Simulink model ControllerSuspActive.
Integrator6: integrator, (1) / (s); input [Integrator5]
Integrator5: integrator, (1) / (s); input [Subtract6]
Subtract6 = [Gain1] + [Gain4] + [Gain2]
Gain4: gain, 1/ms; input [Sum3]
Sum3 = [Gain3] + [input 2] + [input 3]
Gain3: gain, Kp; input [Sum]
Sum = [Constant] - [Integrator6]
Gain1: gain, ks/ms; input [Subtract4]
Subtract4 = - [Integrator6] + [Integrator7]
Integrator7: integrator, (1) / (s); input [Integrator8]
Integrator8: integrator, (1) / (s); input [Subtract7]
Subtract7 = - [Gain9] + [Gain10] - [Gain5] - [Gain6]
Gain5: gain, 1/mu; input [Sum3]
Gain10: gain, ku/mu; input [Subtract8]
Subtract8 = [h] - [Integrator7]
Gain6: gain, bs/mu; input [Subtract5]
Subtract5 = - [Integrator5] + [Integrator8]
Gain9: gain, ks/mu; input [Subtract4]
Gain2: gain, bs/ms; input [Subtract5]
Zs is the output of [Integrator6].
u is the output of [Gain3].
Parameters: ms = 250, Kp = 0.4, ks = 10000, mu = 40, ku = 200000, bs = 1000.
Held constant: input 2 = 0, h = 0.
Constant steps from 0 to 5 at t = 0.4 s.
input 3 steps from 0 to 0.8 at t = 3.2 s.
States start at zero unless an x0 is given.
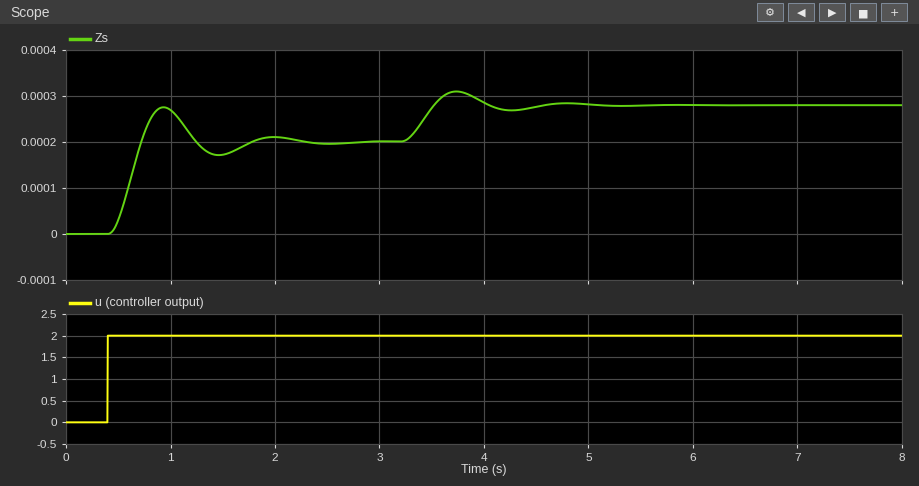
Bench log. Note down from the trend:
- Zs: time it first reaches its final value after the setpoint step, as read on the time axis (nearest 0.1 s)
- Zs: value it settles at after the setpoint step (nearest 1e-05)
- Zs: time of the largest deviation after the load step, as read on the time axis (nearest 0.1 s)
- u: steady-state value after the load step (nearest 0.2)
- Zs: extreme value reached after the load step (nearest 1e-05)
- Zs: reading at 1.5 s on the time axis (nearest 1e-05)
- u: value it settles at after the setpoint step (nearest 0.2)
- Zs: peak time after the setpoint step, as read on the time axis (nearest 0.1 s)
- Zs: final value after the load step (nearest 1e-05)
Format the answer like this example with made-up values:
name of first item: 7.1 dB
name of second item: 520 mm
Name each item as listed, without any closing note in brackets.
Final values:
Zs: time it first reaches its final value after the setpoint step, as read on the time axis: 0.7 s
Zs: value it settles at after the setpoint step: 0.00020
Zs: time of the largest deviation after the load step, as read on the time axis: 3.7 s
u: steady-state value after the load step: 2.0
Zs: extreme value reached after the load step: 0.00031
Zs: reading at 1.5 s on the time axis: 0.00017
u: value it settles at after the setpoint step: 2.0
Zs: peak time after the setpoint step, as read on the time axis: 0.9 s
Zs: final value after the load step: 0.00028
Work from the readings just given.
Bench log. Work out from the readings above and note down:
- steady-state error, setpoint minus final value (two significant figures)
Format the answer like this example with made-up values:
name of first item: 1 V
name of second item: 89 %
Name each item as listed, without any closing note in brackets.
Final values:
steady-state error, setpoint minus final value: 5.0
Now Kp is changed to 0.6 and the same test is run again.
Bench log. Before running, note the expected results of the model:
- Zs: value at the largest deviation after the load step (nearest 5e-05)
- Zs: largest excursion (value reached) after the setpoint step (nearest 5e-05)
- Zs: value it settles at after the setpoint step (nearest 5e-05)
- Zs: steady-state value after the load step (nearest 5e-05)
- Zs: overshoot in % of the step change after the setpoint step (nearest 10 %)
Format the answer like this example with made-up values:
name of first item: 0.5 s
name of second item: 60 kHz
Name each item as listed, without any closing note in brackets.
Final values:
Zs: value at the largest deviation after the load step: 0.00040
Zs: largest excursion (value reached) after the setpoint step: 0.00040
Zs: value it settles at after the setpoint step: 0.00030
Zs: steady-state value after the load step: 0.00040
Zs: overshoot in % of the step change after the setpoint step: 40 %
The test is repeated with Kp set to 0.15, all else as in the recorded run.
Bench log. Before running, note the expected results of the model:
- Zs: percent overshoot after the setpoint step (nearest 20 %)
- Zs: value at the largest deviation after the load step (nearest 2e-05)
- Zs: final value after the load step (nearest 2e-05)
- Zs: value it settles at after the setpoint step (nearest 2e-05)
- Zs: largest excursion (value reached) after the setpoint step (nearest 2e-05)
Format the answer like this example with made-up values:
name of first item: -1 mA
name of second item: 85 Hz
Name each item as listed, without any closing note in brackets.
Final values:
Zs: percent overshoot after the setpoint step: 40 %
Zs: value at the largest deviation after the load step: 0.00018
Zs: final value after the load step: 0.00016
Zs: value it settles at after the setpoint step: 0.00008
Zs: largest excursion (value reached) after the setpoint step: 0.00010
